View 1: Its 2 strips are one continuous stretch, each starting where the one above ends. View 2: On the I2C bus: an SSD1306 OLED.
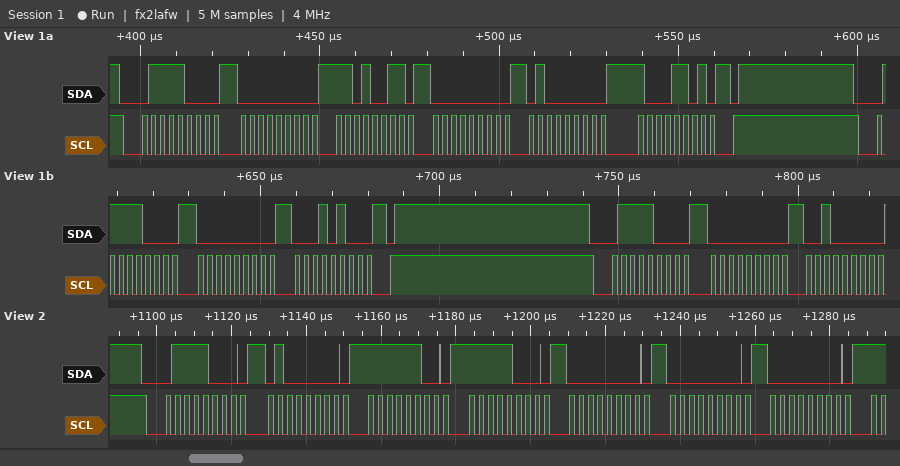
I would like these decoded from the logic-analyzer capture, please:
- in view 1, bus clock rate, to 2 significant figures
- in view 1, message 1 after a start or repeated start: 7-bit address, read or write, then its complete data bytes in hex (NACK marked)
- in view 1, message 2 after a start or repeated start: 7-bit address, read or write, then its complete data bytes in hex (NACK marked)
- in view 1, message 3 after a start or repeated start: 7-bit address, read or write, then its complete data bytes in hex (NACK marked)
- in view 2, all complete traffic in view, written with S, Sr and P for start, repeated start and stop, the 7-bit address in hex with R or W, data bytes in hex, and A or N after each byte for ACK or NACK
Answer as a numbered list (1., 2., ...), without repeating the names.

1. 400 kHz
2. 0x3C write: 00 D3 00 40 8D
3. 0x3C write: 00 14
4. 0x3C write: 00 20
5. S 3CW A 40 A FC A F8 A 00 A 00 A 00 A
